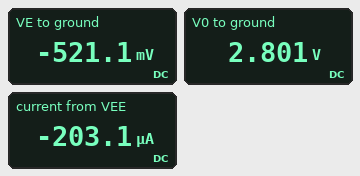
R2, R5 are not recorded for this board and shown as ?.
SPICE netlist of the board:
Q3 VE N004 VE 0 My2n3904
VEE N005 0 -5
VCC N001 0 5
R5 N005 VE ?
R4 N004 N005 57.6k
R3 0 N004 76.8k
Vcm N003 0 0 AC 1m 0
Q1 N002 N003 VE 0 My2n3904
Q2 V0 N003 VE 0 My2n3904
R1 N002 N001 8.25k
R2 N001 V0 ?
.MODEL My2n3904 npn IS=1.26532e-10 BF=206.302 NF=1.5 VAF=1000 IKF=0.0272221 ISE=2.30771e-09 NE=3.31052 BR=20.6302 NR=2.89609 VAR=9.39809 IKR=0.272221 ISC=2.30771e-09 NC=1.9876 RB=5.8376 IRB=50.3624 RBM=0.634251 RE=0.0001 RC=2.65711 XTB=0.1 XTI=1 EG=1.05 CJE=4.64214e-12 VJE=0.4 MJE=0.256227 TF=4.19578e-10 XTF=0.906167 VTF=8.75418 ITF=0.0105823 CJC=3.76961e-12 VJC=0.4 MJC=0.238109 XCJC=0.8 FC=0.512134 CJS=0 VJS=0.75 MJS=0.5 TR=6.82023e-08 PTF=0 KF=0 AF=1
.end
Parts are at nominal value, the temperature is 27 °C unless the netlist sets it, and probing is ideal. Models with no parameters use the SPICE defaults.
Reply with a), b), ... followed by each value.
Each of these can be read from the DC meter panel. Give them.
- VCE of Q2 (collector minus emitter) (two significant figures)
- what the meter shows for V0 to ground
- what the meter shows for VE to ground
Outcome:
a) 3.3 V
b) 2.801 V
c) -521.1 mV
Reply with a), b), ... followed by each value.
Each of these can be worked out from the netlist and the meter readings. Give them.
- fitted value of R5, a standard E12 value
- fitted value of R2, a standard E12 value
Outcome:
a) 27 kΩ
b) 27 kΩ
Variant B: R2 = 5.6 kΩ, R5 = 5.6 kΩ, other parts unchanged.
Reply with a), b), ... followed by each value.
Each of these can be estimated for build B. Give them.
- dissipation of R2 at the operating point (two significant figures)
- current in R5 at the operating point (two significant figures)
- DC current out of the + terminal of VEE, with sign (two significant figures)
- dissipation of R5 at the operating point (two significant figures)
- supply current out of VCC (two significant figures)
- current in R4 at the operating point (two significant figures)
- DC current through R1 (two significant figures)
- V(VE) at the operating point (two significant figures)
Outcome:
a) 850 µW
b) 790 µA
c) -830 µA
d) 3.5 mW
e) 780 µA
f) 37 µA
g) 390 µA
h) -580 mV
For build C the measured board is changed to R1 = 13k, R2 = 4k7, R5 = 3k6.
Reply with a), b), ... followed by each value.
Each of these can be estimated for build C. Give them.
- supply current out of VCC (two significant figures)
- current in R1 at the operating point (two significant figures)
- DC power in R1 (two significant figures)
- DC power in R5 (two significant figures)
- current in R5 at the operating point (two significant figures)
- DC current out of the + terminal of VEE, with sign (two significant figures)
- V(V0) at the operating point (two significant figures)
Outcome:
a) 1.0 mA
b) 430 µA
c) 2.4 mW
d) 5.4 mW
e) 1.2 mA
f) -1.3 mA
g) 2.1 V
